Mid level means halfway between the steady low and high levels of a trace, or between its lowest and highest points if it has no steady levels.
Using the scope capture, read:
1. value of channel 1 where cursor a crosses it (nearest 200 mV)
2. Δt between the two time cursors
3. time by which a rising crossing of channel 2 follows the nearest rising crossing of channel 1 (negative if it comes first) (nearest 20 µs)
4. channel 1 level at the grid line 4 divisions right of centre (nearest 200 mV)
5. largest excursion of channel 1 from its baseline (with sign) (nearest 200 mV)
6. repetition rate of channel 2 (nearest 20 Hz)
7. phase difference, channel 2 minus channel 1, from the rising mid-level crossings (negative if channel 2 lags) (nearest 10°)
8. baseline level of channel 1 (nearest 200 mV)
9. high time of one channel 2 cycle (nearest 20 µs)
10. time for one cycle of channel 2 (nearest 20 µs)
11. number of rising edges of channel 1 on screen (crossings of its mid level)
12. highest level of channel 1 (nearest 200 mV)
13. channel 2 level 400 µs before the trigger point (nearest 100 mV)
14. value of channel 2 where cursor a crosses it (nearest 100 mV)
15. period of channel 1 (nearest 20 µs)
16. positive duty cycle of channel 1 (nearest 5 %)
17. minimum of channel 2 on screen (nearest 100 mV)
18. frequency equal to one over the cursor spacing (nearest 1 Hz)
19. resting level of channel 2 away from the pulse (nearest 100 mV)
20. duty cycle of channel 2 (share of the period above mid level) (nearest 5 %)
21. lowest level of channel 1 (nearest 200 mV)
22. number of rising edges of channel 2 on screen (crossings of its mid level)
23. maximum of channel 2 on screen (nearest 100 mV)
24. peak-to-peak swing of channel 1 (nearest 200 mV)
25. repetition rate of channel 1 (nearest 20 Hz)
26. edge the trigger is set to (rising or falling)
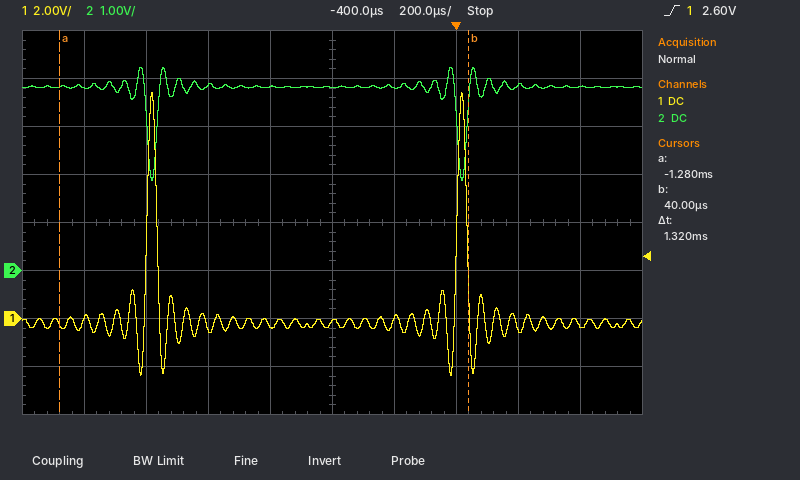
-200 mV
1.32 ms
+40 µs
-200 mV
+9.6 V
1.00 kHz
-10°
-200 mV
960 µs
1.00 ms
2
9.4 V
3.8 V
3.8 V
1.00 ms
5 %
1.9 V
758 Hz
3.8 V
95 %
-2.4 V
2
4.2 V
11.8 V
1.00 kHz
rising
